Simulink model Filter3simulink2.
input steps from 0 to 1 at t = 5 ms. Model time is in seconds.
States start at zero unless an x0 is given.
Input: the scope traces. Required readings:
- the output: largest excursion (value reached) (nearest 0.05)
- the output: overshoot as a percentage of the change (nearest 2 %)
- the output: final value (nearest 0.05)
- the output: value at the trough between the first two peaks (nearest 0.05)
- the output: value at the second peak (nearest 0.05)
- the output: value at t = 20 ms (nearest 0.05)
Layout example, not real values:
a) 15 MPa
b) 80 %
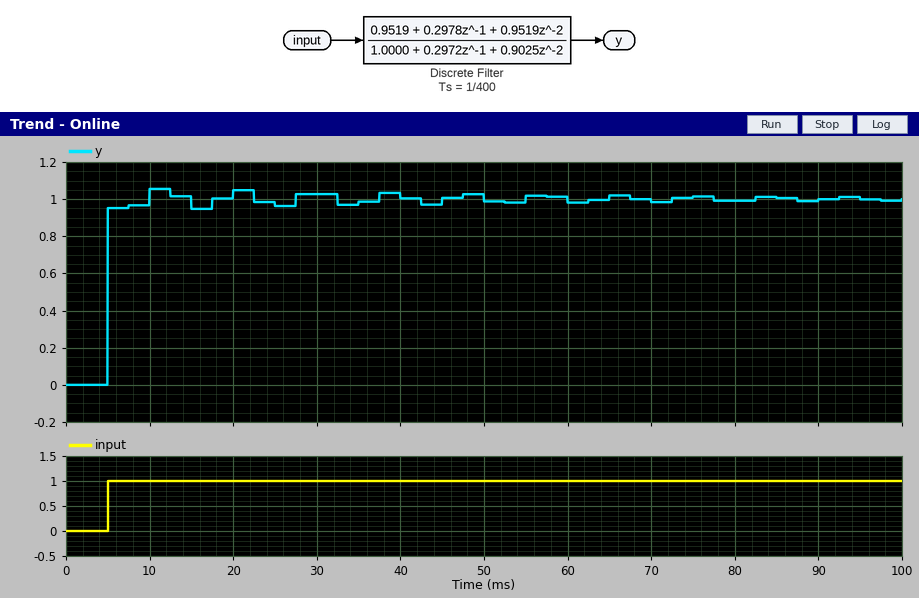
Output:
a) 1.05
b) 6 %
c) 1.00
d) 0.95
e) 1.05
f) 1.05
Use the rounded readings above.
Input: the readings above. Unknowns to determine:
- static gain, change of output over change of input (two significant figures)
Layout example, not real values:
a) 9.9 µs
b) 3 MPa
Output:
a) 1.0
